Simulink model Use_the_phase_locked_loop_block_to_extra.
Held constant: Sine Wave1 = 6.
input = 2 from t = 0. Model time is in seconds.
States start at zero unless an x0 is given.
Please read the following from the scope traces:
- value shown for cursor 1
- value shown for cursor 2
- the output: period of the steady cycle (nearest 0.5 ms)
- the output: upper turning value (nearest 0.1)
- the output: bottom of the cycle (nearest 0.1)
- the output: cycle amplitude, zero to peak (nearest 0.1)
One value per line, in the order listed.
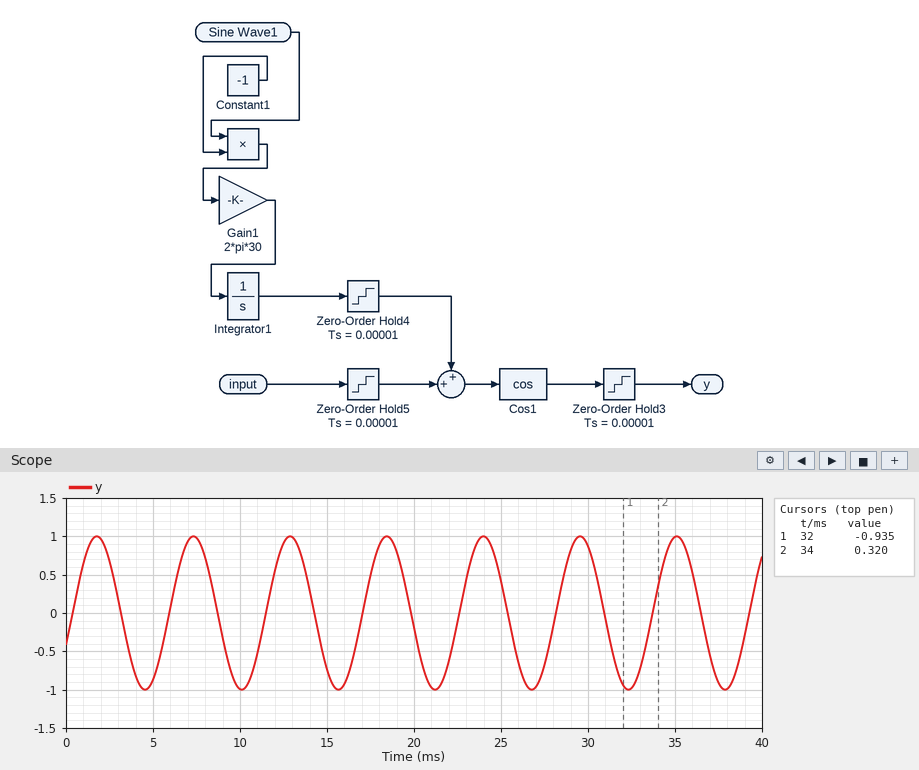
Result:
-0.935
0.320
5.5 ms
1.0
-1.0
1.0
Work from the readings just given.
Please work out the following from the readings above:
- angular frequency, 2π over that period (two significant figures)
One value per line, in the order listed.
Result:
1.1 rad/ms
